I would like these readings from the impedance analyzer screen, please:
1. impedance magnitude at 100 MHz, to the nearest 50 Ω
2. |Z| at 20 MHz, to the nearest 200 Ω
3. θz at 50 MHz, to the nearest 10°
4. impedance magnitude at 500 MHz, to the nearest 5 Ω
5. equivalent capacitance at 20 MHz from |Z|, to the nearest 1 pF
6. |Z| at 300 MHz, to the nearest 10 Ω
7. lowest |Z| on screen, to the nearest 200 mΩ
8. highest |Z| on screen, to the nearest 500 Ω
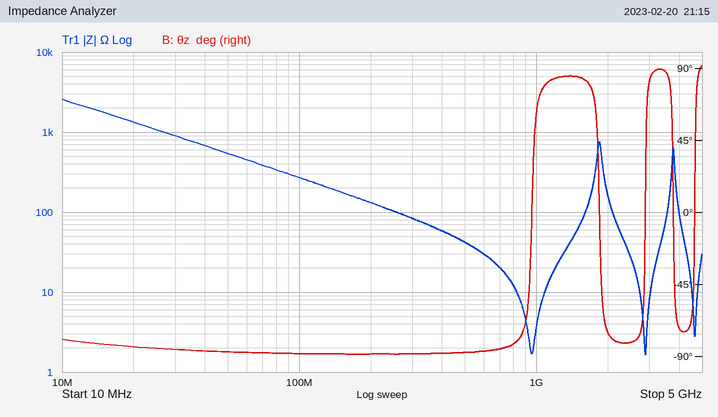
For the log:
250 Ω
1.4 kΩ
-90°
40 Ω
6 pF
80 Ω
1.6 Ω
2.5 kΩ
